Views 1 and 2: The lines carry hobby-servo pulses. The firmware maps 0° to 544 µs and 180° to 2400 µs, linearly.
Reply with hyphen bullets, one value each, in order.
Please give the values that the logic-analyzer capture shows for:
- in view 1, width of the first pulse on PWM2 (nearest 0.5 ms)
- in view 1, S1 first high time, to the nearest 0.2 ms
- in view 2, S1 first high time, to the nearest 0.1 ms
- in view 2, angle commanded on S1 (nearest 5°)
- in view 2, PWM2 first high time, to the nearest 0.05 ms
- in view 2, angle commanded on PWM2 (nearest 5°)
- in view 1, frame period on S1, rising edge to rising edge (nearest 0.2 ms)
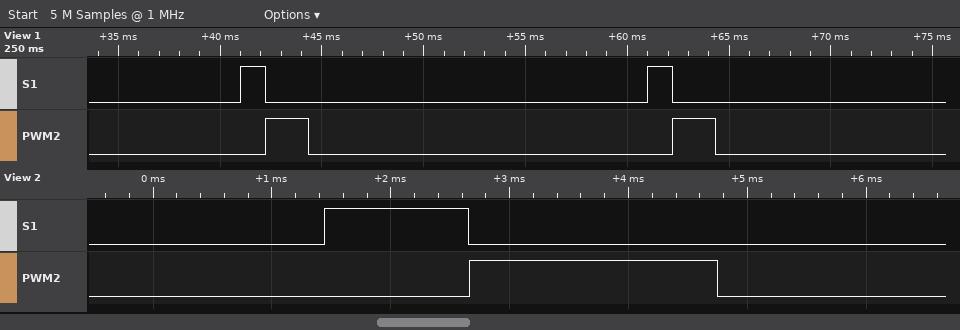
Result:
- 2.0 ms
- 1.2 ms
- 1.2 ms
- 65°
- 2.10 ms
- 150°
- 20.0 ms
